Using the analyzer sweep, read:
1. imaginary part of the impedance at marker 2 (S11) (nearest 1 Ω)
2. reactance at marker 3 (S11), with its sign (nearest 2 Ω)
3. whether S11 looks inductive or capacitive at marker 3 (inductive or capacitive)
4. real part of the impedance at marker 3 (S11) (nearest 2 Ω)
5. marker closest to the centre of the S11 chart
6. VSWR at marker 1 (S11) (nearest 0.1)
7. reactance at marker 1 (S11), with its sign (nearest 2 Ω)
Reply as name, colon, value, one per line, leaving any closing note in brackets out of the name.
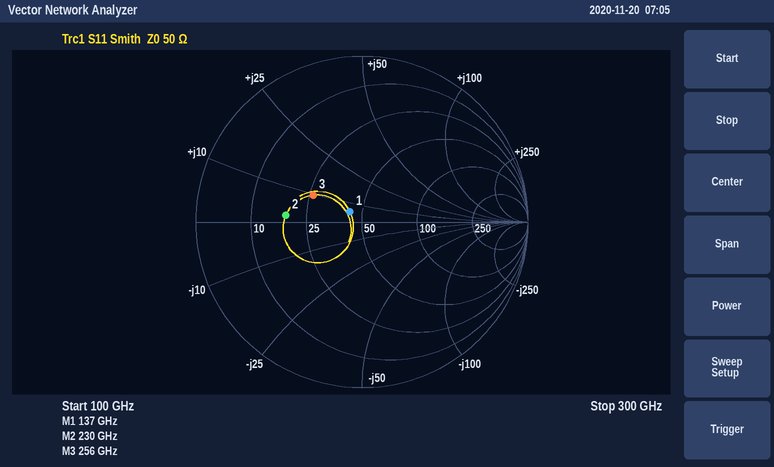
imaginary part of the impedance at marker 2 (S11): +2 Ω
reactance at marker 3 (S11), with its sign: +10 Ω
whether S11 looks inductive or capacitive at marker 3: inductive
real part of the impedance at marker 3 (S11): 26 Ω
marker closest to the centre of the S11 chart: marker 1
VSWR at marker 1 (S11): 1.2
reactance at marker 1 (S11), with its sign: +6 Ω
